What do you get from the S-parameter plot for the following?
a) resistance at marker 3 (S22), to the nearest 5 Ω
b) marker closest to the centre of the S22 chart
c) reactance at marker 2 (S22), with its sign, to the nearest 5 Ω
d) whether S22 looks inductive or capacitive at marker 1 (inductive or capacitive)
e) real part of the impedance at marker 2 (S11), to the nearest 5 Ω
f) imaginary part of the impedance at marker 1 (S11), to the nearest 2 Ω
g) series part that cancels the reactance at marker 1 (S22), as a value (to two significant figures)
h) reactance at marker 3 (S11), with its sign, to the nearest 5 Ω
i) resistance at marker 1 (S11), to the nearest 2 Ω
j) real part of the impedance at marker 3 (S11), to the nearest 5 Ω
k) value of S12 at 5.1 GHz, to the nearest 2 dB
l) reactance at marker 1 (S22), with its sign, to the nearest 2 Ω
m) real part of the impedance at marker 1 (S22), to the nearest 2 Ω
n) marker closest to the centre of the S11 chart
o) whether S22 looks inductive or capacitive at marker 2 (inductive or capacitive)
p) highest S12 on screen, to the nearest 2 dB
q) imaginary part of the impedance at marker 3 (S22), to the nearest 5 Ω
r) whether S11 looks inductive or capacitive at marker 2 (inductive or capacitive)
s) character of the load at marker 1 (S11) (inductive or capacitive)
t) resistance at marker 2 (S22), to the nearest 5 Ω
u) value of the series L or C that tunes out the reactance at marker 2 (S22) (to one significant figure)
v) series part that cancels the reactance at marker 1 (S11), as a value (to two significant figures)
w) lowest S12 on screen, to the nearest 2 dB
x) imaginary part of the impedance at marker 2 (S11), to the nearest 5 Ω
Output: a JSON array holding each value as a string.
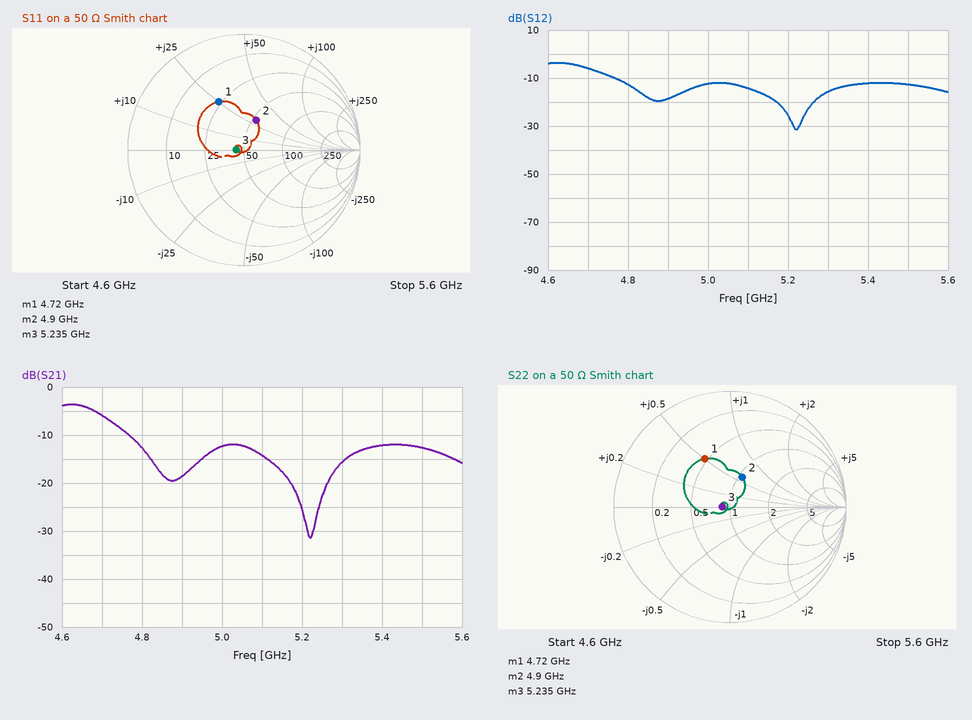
["45 Ω", "marker 3", "+30 Ω", "inductive", "55 Ω", "+26 Ω", "1.3 pF", "0 Ω", "24 Ω", "45 Ω", "-14 dB", "+26 Ω", "24 Ω", "marker 3", "inductive", "-4 dB", "0 Ω", "inductive", "inductive", "55 Ω", "1 pF", "1.3 pF", "-32 dB", "+30 Ω"]
